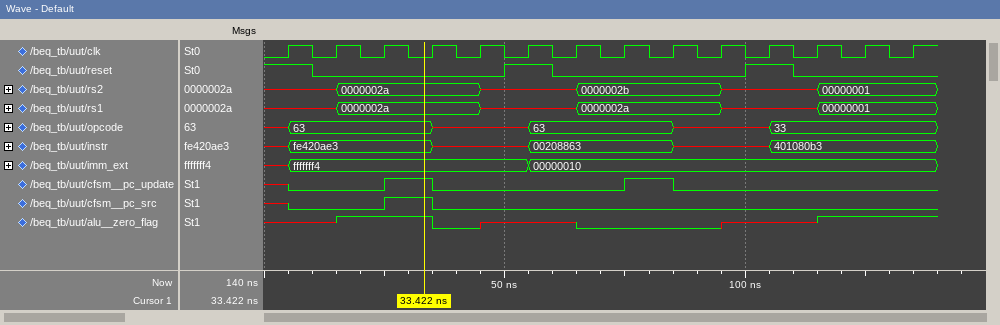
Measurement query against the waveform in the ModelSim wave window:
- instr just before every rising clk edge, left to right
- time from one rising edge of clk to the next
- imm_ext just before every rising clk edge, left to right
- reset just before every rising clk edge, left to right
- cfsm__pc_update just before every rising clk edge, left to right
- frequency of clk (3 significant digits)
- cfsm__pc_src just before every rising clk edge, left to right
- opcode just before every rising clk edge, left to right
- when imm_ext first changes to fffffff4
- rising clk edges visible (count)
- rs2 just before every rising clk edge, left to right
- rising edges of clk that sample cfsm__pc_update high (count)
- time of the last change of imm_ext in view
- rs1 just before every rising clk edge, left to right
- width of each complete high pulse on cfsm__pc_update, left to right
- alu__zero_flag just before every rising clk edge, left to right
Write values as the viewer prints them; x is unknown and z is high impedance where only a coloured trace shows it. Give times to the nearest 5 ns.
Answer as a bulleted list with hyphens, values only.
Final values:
- x, fe420ae3, fe420ae3, fe420ae3, x, x, 00208863, 00208863, 00208863, x, x, 401080b3, 401080b3, 401080b3
- 10 ns
- x, fffffff4, fffffff4, fffffff4, fffffff4, fffffff4, 00000010, 00000010, 00000010, 00000010, 00000010, 00000010, 00000010, 00000010
- 1 0 0 0 0 1 0 0 0 0 1 0 0 0
- x 0 0 1 0 0 0 0 1 0 0 0 0 0
- 100 MHz
- x 0 0 1 0 0 0 0 0 0 0 0 0 0
- x, 63, 63, 63, x, x, 63, 63, 63, x, x, 33, 33, 33
- 5 ns
- 14
- x, x, 0000002a, 0000002a, 0000002a, x, x, 0000002b, 0000002b, 0000002b, x, x, 00000001, 00000001
- 2
- 55 ns
- x, x, 0000002a, 0000002a, 0000002a, x, x, 0000002a, 0000002a, 0000002a, x, x, 00000001, 00000001
- 10 ns, 10 ns
- x x 1 1 0 x x 0 0 0 x x 1 1
